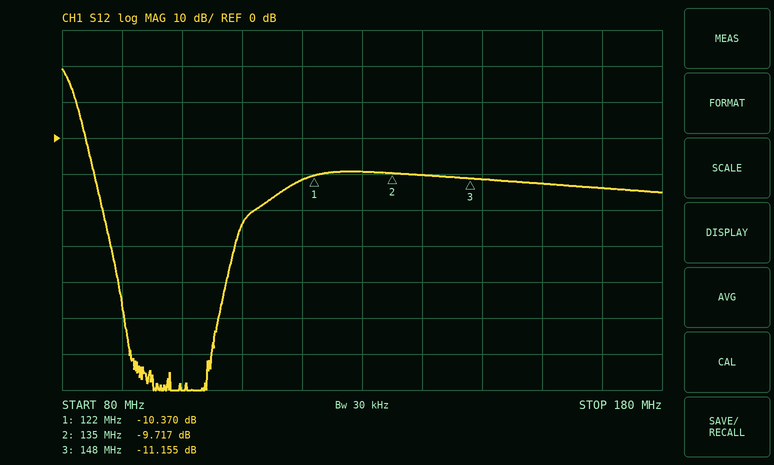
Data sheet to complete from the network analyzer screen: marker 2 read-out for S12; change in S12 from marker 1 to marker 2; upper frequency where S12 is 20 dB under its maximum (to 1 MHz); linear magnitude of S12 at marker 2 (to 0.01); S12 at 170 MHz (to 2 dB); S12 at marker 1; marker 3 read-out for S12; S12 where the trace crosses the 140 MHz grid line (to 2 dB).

-9.717 dB
0.653 dB
84 MHz
0.33
-14 dB
-10.370 dB
-11.155 dB
-10 dB
